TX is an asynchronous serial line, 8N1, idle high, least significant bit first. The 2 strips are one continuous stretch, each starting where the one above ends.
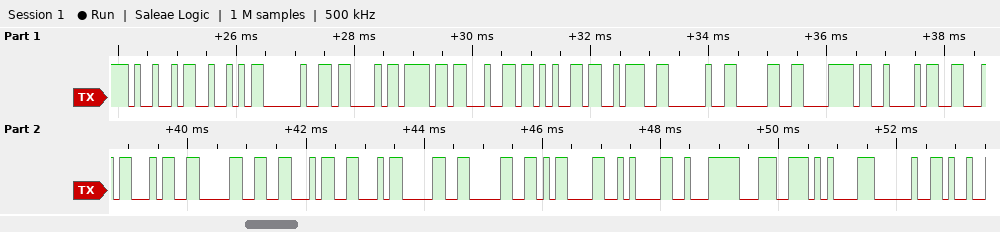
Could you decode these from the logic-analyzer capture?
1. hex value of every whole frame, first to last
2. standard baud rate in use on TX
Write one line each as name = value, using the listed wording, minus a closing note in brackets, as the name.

hex value of every whole frame, first to last = 49 52 20 43 6F 64 65 3A 20 30 78 42 46 34 30 46 46 30 30 0D 0A E2 9C 85 20
standard baud rate in use on TX = 9600 baud
